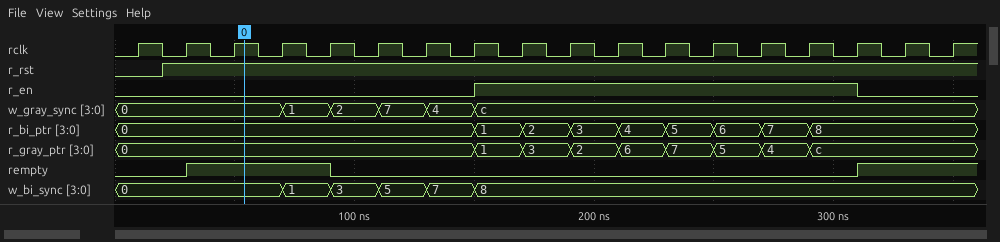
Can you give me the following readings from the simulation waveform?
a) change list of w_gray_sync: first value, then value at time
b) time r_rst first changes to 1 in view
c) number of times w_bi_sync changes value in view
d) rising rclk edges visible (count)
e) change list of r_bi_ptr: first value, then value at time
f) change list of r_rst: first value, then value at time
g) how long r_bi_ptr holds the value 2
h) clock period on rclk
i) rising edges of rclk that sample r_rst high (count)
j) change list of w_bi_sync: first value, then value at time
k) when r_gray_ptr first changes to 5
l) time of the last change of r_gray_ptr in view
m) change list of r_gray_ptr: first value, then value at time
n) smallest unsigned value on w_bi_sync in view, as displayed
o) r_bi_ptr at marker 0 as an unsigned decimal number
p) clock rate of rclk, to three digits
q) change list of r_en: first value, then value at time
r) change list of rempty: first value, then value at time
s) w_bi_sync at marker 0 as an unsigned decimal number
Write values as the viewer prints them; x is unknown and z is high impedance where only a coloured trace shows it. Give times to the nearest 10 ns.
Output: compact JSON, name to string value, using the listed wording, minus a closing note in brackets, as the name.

{"change list of w_gray_sync: first value, then value at time": "0, 1 at 70 ns, 2 at 90 ns, 7 at 110 ns, 4 at 130 ns, c at 150 ns", "time r_rst first changes to 1 in view": "20 ns", "number of times w_bi_sync changes value in view": "5", "rising rclk edges visible": "18", "change list of r_bi_ptr: first value, then value at time": "0, 1 at 150 ns, 2 at 170 ns, 3 at 190 ns, 4 at 210 ns, 5 at 230 ns, 6 at 250 ns, 7 at 270 ns, 8 at 290 ns", "change list of r_rst: first value, then value at time": "0, 1 at 20 ns", "how long r_bi_ptr holds the value 2": "20 ns", "clock period on rclk": "20 ns", "rising edges of rclk that sample r_rst high": "17", "change list of w_bi_sync: first value, then value at time": "0, 1 at 70 ns, 3 at 90 ns, 5 at 110 ns, 7 at 130 ns, 8 at 150 ns", "when r_gray_ptr first changes to 5": "250 ns", "time of the last change of r_gray_ptr in view": "290 ns", "change list of r_gray_ptr: first value, then value at time": "0, 1 at 150 ns, 3 at 170 ns, 2 at 190 ns, 6 at 210 ns, 7 at 230 ns, 5 at 250 ns, 4 at 270 ns, c at 290 ns", "smallest unsigned value on w_bi_sync in view, as displayed": "0", "r_bi_ptr at marker 0 as an unsigned decimal number": "0", "clock rate of rclk, to three digits": "50.0 MHz", "change list of r_en: first value, then value at time": "0, 1 at 150 ns, 0 at 310 ns", "change list of rempty: first value, then value at time": "0, 1 at 30 ns, 0 at 90 ns, 1 at 310 ns", "w_bi_sync at marker 0 as an unsigned decimal number": "0"}
